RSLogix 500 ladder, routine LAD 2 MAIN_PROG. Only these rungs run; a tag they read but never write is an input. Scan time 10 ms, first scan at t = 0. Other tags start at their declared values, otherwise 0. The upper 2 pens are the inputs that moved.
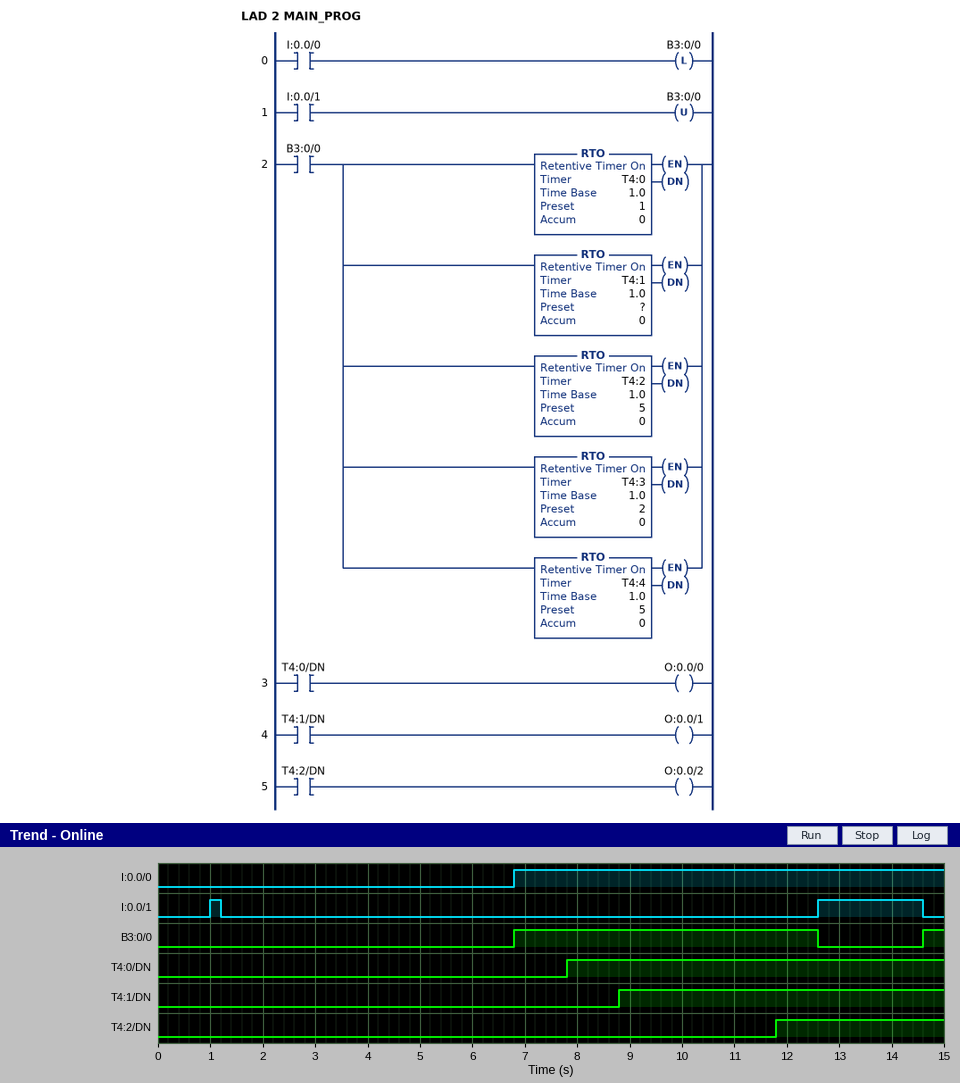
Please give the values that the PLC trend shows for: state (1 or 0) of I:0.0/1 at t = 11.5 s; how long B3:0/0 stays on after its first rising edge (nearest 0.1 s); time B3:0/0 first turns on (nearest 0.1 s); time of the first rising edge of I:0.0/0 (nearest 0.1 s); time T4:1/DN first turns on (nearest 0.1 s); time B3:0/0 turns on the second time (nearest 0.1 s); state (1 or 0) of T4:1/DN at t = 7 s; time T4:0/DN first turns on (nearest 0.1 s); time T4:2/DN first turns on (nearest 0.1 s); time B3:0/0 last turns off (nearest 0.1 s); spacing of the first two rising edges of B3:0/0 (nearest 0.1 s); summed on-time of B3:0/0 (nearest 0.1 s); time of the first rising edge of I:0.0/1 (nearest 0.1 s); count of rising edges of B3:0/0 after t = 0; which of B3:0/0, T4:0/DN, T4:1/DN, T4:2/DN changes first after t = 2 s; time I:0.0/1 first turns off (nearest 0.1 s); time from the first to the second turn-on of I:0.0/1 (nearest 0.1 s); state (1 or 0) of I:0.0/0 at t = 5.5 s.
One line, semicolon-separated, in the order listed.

0; 5.8 s; 6.8 s; 6.8 s; 8.8 s; 14.6 s; 0; 7.8 s; 11.8 s; 12.6 s; 7.8 s; 6.2 s; 1.0 s; 2; B3:0/0; 1.2 s; 11.6 s; 0
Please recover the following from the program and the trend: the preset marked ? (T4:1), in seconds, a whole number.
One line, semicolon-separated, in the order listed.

2 s
